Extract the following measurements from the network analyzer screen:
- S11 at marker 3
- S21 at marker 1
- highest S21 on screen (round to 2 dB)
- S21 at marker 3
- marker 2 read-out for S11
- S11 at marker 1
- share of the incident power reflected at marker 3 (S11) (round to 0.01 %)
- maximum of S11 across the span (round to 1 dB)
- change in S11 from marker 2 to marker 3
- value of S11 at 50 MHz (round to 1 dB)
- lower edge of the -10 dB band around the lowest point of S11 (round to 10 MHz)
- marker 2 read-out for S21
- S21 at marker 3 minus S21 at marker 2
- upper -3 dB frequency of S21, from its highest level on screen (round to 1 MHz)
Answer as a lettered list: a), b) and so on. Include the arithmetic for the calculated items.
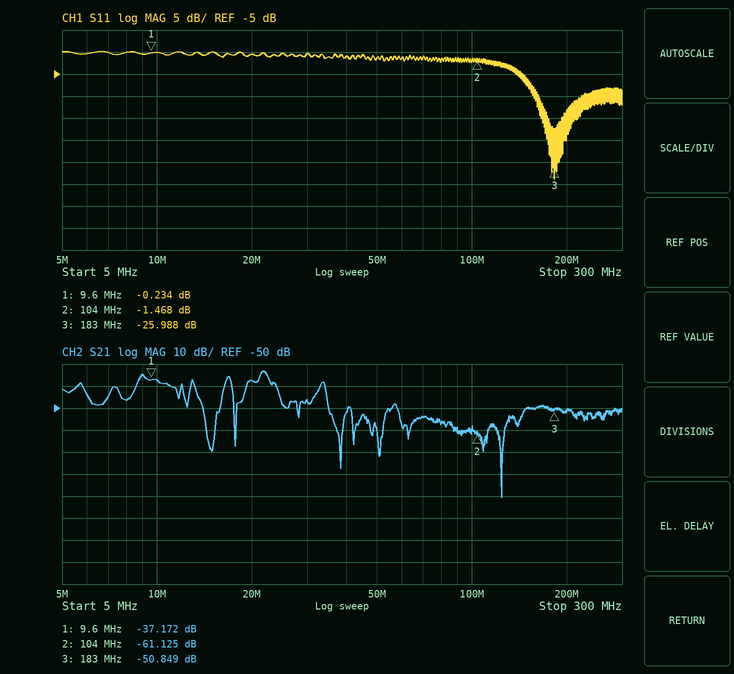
a) -25.988 dB
b) -37.172 dB
c) -34 dB
d) -50.849 dB
e) -1.468 dB
f) -0.234 dB
g) 10^(-25.988/10) ≈ 0.25 %
h) 0 dB
i) -25.988 − (-1.468) = -24.520 dB
j) -1 dB
k) 160 MHz
l) -61.125 dB
m) -50.849 − (-61.125) = 10.276 dB
n) 23 MHz
